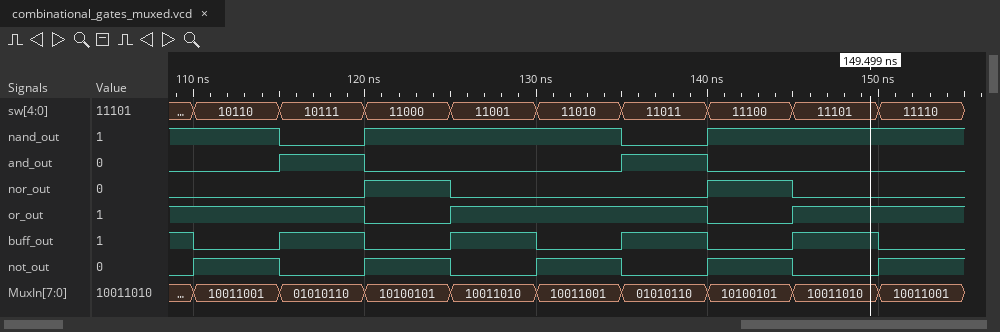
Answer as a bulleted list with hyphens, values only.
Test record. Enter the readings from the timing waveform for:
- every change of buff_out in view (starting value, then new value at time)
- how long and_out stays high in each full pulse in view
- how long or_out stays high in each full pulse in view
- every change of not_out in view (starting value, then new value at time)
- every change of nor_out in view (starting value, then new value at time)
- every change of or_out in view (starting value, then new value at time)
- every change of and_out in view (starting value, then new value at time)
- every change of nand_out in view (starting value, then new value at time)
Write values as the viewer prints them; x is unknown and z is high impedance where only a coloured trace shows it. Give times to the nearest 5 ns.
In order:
- 1, 0 at 110 ns, 1 at 115 ns, 0 at 120 ns, 1 at 125 ns, 0 at 130 ns, 1 at 135 ns, 0 at 140 ns, 1 at 145 ns, 0 at 150 ns
- 5 ns, 5 ns
- 15 ns
- 0, 1 at 110 ns, 0 at 115 ns, 1 at 120 ns, 0 at 125 ns, 1 at 130 ns, 0 at 135 ns, 1 at 140 ns, 0 at 145 ns, 1 at 150 ns
- 0, 1 at 120 ns, 0 at 125 ns, 1 at 140 ns, 0 at 145 ns
- 1, 0 at 120 ns, 1 at 125 ns, 0 at 140 ns, 1 at 145 ns
- 0, 1 at 115 ns, 0 at 120 ns, 1 at 135 ns, 0 at 140 ns
- 1, 0 at 115 ns, 1 at 120 ns, 0 at 135 ns, 1 at 140 ns
